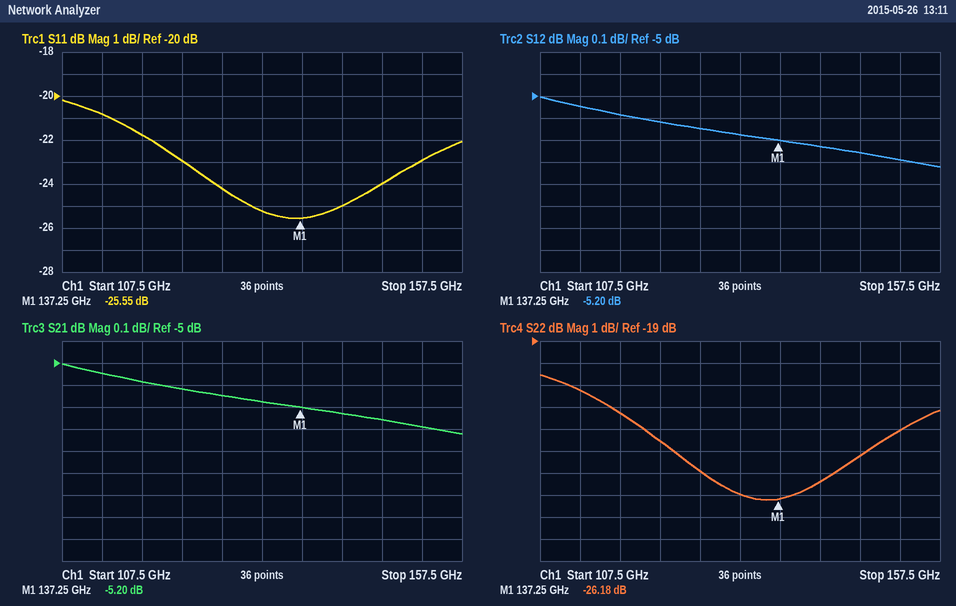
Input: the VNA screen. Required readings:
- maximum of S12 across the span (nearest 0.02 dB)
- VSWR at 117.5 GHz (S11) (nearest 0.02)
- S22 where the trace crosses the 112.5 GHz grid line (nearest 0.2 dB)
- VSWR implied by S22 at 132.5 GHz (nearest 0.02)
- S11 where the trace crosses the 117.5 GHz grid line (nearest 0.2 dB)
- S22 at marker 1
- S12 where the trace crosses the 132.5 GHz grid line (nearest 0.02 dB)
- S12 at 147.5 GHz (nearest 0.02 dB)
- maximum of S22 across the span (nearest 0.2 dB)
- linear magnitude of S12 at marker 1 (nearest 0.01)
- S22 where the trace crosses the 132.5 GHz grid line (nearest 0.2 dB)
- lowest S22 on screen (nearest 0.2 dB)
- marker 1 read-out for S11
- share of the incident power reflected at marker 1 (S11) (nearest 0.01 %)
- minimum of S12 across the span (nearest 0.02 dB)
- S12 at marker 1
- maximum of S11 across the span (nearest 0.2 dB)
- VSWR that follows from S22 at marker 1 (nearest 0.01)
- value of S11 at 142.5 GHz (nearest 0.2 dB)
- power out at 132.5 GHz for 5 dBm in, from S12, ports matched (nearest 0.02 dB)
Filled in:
-5.00 dB
1.18
-21.2 dB
1.10
-21.8 dB
-26.18 dB
-5.18 dB
-5.26 dB
-20.6 dB
0.55
-26.0 dB
-26.2 dB
-25.55 dB
0.28 %
-5.32 dB
-5.20 dB
-20.2 dB
1.10
-25.0 dB
-0.18 dBm
